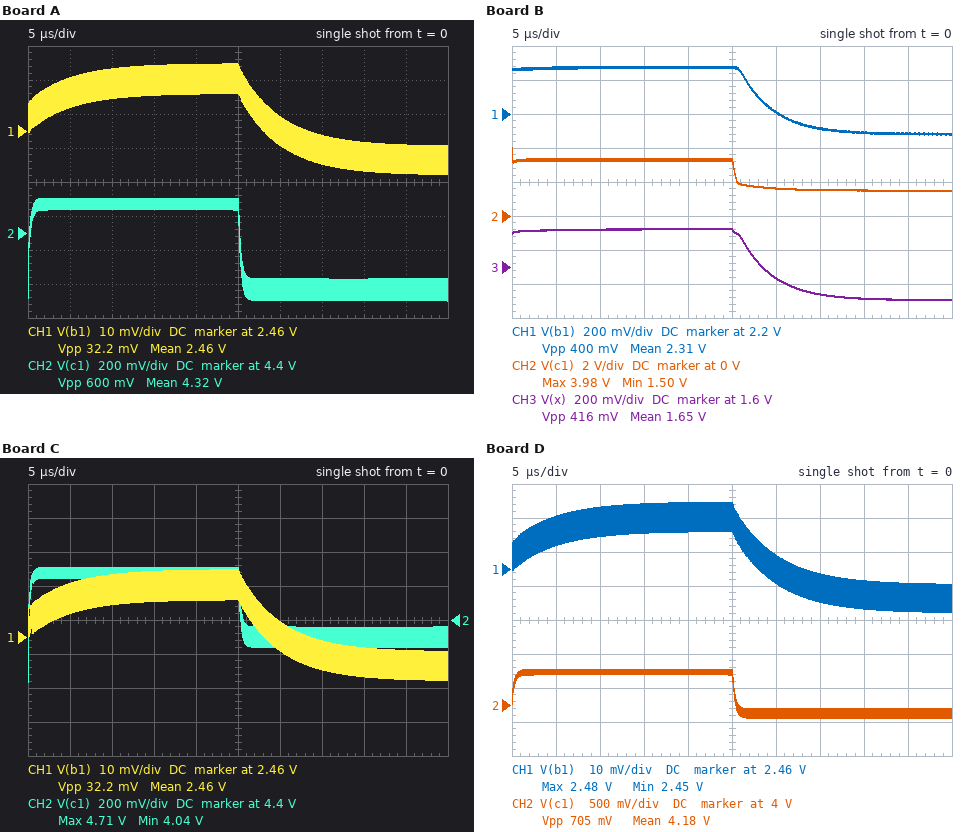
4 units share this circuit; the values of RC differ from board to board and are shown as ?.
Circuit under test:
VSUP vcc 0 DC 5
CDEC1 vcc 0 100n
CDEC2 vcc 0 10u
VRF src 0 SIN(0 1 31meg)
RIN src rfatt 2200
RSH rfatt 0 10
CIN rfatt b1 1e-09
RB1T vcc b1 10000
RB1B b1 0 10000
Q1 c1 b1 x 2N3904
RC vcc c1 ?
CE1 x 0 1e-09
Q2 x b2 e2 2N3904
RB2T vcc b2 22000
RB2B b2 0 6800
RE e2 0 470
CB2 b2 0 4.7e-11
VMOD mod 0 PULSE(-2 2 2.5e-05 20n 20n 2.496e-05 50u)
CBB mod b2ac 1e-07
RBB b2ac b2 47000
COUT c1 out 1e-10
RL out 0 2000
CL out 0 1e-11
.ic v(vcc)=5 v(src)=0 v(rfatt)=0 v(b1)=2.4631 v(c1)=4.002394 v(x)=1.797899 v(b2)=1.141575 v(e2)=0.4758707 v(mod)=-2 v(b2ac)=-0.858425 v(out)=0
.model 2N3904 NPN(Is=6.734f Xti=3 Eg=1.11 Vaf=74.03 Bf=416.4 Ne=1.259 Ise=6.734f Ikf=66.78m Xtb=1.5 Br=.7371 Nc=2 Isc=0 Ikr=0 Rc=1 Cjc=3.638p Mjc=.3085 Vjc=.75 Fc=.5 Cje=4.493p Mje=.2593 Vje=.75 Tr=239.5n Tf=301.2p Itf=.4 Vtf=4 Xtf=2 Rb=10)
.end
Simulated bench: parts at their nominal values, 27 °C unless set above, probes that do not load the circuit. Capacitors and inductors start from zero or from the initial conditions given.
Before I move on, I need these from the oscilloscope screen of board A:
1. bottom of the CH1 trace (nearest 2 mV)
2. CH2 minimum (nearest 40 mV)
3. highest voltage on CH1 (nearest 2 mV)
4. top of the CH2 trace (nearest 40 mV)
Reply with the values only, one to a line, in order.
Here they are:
2.448 V
4.00 V
2.480 V
4.60 V
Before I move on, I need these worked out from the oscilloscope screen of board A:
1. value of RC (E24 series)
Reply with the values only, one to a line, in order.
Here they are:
680 Ω
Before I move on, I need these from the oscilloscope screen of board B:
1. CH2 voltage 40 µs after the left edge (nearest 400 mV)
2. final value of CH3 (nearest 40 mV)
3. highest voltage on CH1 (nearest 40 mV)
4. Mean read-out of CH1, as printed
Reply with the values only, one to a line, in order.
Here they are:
1.6 V
1.40 V
2.48 V
2.31 V
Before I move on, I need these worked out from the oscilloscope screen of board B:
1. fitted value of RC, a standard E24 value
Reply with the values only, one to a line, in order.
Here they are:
2.7 kΩ
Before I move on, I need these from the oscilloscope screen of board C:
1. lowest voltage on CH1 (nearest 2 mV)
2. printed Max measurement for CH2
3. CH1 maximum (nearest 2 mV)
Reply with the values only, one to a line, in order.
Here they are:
2.448 V
4.71 V
2.480 V
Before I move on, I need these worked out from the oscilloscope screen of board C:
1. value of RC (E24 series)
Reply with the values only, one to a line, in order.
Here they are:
510 Ω
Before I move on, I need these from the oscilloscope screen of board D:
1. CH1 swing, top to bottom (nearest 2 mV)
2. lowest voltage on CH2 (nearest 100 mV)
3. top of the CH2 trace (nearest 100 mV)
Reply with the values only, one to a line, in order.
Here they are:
32 mV
3.8 V
4.5 V
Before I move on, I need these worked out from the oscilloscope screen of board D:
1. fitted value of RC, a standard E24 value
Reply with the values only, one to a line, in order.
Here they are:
820 Ω
